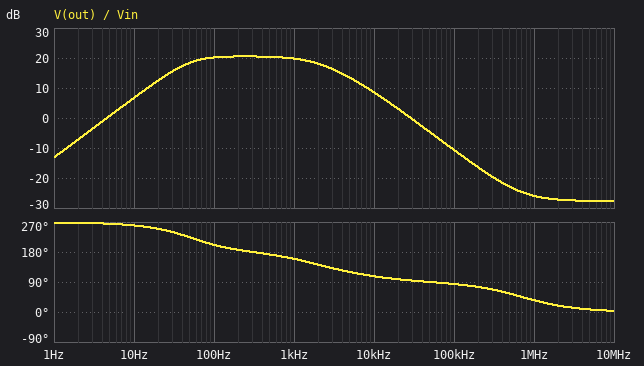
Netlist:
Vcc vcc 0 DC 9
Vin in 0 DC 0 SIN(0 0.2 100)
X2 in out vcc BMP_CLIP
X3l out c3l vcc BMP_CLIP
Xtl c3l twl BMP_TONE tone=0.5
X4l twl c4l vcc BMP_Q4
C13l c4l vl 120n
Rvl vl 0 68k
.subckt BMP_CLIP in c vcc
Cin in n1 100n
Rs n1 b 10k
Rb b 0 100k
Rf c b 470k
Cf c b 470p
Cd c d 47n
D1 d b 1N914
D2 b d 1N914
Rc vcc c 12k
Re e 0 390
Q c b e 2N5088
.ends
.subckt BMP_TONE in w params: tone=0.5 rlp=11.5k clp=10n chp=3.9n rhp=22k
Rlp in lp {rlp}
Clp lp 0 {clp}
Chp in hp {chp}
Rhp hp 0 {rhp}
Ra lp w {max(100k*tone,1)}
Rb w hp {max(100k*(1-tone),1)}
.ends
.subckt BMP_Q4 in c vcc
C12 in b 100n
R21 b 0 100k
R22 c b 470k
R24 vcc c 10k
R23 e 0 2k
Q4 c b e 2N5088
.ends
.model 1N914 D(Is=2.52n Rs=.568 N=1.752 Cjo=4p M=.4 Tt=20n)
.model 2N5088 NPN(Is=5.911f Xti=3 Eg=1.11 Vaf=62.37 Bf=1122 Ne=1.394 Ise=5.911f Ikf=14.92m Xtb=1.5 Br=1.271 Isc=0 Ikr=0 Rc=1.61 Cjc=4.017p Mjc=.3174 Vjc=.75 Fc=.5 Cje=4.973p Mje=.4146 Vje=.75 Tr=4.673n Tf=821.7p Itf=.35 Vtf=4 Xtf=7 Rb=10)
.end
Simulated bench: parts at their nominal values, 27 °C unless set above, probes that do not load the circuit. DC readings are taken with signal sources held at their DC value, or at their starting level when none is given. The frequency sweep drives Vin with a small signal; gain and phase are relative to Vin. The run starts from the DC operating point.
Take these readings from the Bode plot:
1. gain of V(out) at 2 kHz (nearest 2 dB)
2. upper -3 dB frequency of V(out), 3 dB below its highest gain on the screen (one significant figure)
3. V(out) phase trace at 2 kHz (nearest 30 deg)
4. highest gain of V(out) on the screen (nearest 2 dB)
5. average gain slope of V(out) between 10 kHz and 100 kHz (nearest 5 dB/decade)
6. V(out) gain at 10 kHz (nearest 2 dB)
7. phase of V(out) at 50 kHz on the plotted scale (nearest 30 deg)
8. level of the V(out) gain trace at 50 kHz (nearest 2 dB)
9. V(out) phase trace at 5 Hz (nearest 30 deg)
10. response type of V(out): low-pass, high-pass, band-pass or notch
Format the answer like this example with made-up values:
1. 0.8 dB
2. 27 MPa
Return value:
1. 18 dB
2. 2 kHz
3. 150 deg
4. 20 dB
5. -20 dB/decade
6. 8 dB
7. 90 deg
8. -4 dB
9. 270 deg
10. band-pass
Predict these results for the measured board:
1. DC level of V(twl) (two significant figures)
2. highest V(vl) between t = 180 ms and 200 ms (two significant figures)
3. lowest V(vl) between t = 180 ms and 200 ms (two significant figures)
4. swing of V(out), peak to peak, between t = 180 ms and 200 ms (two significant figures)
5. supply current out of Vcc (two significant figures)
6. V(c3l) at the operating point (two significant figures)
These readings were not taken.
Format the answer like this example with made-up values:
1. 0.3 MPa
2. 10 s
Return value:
1. 2.5 V
2. 1.1 V
3. -1.1 V
4. 1.1 V
5. 970 µA
6. 4.6 V
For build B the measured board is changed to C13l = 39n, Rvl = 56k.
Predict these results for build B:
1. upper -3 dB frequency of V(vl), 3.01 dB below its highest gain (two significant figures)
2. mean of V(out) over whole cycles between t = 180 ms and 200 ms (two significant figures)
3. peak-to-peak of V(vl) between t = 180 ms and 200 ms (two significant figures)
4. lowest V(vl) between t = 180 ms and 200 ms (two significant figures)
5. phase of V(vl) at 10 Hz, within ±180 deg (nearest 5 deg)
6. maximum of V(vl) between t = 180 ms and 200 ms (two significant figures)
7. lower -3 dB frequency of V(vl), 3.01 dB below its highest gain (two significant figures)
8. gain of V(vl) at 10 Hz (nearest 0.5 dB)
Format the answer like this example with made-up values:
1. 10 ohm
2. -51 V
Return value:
1. 820 Hz
2. 4.7 V
3. 1.7 V
4. -870 mV
5. 125 deg
6. 870 mV
7. 91 Hz
8. -8.5 dB
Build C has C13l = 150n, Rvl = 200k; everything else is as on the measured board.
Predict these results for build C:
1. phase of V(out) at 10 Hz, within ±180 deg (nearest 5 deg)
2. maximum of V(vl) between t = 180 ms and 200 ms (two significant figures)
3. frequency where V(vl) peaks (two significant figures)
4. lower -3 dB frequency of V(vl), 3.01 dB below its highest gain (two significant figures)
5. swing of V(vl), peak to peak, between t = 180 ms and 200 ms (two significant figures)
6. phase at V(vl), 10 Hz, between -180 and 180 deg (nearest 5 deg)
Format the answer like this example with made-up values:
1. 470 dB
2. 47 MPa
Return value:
1. -100 deg
2. 1.2 V
3. 220 Hz
4. 71 Hz
5. 2.5 V
6. 70 deg
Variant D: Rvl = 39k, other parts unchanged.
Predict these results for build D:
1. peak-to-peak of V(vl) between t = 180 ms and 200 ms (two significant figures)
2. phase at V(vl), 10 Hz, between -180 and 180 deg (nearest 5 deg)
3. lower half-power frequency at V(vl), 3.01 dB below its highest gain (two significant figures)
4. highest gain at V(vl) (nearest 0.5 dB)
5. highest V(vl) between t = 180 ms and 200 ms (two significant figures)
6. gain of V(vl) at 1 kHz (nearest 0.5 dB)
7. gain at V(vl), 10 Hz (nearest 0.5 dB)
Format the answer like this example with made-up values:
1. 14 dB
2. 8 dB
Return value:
1. 1.9 V
2. 115 deg
3. 76 Hz
4. 43.5 dB
5. 950 mV
6. 39.0 dB
7. -2.0 dB
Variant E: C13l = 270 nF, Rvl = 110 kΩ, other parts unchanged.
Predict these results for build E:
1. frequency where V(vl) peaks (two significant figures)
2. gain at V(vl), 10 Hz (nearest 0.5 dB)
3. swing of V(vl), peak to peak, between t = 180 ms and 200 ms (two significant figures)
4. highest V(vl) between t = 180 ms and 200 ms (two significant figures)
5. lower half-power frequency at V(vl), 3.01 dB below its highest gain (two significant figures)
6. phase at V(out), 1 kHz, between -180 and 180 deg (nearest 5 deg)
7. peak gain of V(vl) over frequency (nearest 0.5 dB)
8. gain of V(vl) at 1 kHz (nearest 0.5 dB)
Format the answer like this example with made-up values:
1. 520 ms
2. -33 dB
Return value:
1. 220 Hz
2. 7.5 dB
3. 2.4 V
4. 1.2 V
5. 71 Hz
6. 160 deg
7. 44.5 dB
8. 40.0 dB
